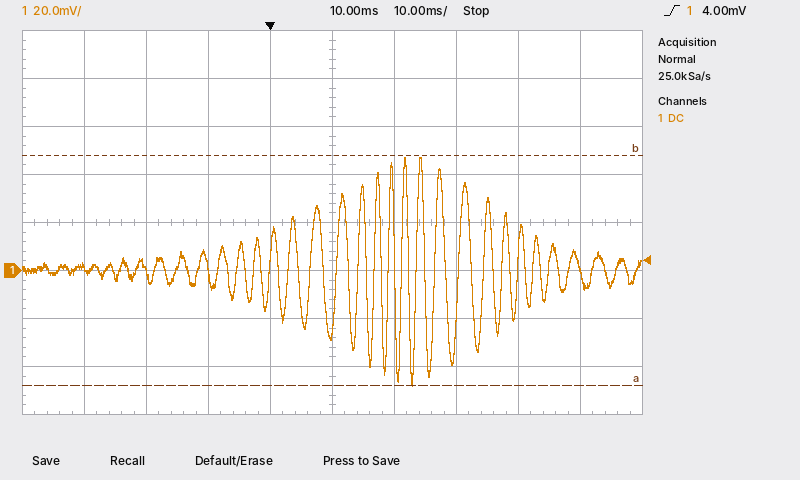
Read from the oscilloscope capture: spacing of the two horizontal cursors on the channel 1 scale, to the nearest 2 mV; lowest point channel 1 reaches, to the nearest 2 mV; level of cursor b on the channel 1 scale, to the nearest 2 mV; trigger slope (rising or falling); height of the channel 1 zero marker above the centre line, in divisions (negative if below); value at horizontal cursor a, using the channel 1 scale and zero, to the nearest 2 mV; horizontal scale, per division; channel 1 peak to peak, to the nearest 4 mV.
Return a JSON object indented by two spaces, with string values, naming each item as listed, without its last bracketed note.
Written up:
{
  "spacing of the two horizontal cursors on the channel 1 scale, to the nearest 2 mV": "96 mV",
  "lowest point channel 1 reaches, to the nearest 2 mV": "-48 mV",
  "level of cursor b on the channel 1 scale, to the nearest 2 mV": "48 mV",
  "trigger slope": "rising",
  "height of the channel 1 zero marker above the centre line, in divisions": "-1.0 div",
  "value at horizontal cursor a, using the channel 1 scale and zero, to the nearest 2 mV": "-48 mV",
  "horizontal scale, per division": "10 ms",
  "channel 1 peak to peak, to the nearest 4 mV": "96 mV"
}
